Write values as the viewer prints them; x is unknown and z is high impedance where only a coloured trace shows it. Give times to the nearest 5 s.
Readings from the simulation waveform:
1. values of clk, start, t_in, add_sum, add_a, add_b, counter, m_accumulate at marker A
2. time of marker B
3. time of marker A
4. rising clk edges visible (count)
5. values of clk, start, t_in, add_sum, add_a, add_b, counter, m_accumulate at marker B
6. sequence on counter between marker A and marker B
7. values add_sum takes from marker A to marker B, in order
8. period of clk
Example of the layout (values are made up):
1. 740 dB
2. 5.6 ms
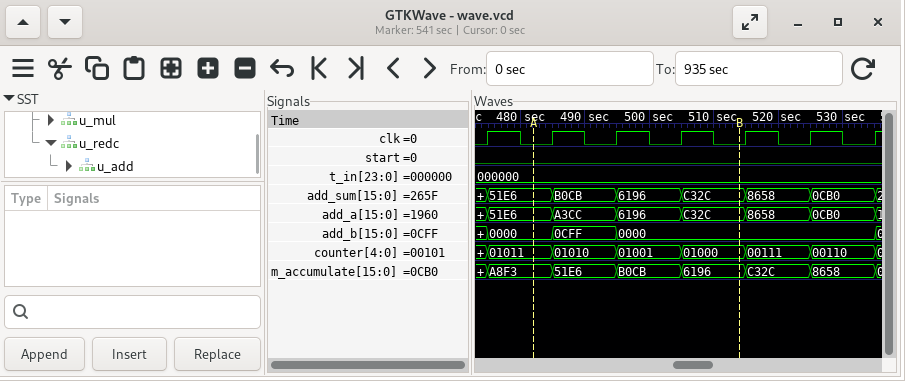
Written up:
1. clk=0, start=0, t_in=000000, add_sum=51E6, add_a=51E6, add_b=0000, counter=01011, m_accumulate=A8F3
2. 515 s
3. 480 s
4. 7
5. clk=0, start=0, t_in=000000, add_sum=C32C, add_a=C32C, add_b=0000, counter=01000, m_accumulate=6196
6. 01011, 01010, 01001, 01000
7. 51E6, B0CB, 6196, C32C
8. 10 s
